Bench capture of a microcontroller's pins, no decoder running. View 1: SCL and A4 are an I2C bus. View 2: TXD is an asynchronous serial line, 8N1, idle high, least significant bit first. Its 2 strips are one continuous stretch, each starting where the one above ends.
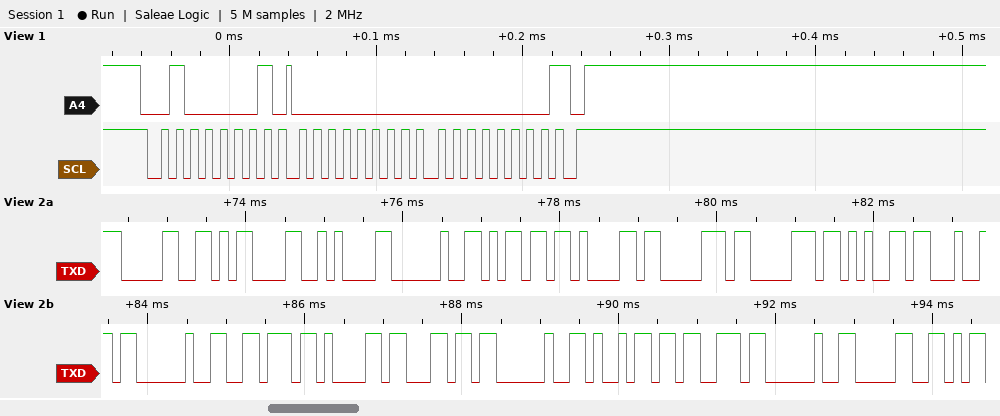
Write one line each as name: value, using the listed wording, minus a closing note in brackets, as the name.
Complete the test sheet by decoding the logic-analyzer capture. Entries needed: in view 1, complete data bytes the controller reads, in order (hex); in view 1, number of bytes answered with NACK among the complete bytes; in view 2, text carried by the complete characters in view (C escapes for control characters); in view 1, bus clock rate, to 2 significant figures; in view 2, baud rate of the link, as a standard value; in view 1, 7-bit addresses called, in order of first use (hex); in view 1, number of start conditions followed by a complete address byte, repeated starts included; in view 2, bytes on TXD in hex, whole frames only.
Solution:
in view 1, complete data bytes the controller reads, in order: 00 00
in view 1, number of bytes answered with NACK among the complete bytes: 1
in view 2, text carried by the complete characters in view: "0\r\n mapped val is 0"
in view 1, bus clock rate, to 2 significant figures: 100 kHz
in view 2, baud rate of the link, as a standard value: 9600 baud
in view 1, 7-bit addresses called, in order of first use: 0x20
in view 1, number of start conditions followed by a complete address byte, repeated starts included: 1
in view 2, bytes on TXD in hex, whole frames only: 0x30 0x0D 0x0A 0x20 0x6D 0x61 0x70 0x70 0x65 0x64 0x20 0x76 0x61 0x6C 0x20 0x69 0x73 0x20 0x30
